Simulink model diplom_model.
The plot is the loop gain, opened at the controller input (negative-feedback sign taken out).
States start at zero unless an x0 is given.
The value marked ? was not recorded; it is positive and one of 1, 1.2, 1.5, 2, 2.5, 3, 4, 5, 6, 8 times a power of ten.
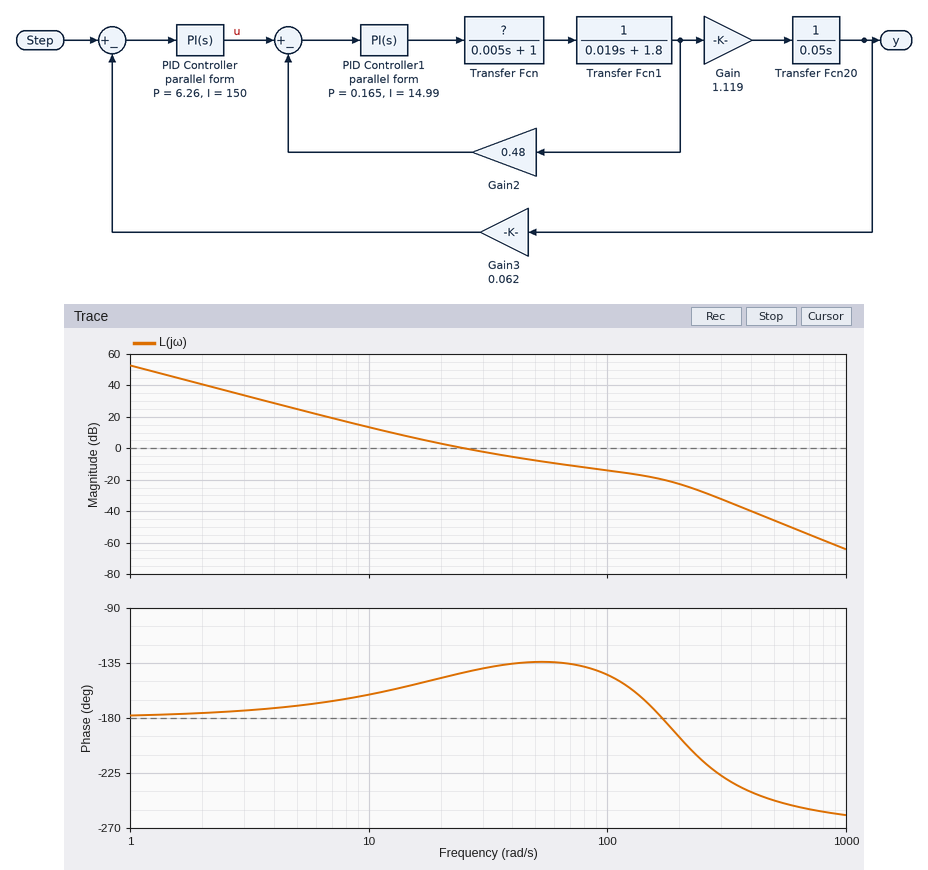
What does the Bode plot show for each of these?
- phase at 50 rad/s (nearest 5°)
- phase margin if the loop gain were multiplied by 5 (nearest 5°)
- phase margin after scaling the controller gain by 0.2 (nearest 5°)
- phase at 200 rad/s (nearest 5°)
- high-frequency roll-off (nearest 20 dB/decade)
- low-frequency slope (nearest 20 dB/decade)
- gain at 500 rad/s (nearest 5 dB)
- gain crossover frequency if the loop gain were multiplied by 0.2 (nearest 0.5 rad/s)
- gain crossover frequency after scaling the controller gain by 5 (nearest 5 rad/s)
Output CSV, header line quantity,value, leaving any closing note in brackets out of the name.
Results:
quantity,value
phase at 50 rad/s,-135°
phase margin if the loop gain were multiplied by 5,35°
phase margin after scaling the controller gain by 0.2,20°
phase at 200 rad/s,-195°
high-frequency roll-off,-60 dB/decade
low-frequency slope,-40 dB/decade
gain at 500 rad/s,-45 dB
gain crossover frequency if the loop gain were multiplied by 0.2,9.5 rad/s
gain crossover frequency after scaling the controller gain by 5,100 rad/s
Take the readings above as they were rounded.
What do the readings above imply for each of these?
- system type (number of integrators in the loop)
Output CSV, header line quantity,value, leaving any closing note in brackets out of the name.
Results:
quantity,value
system type,2
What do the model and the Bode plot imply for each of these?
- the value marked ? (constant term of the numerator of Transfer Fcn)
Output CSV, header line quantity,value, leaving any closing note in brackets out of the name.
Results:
quantity,value
the value marked ?,40
